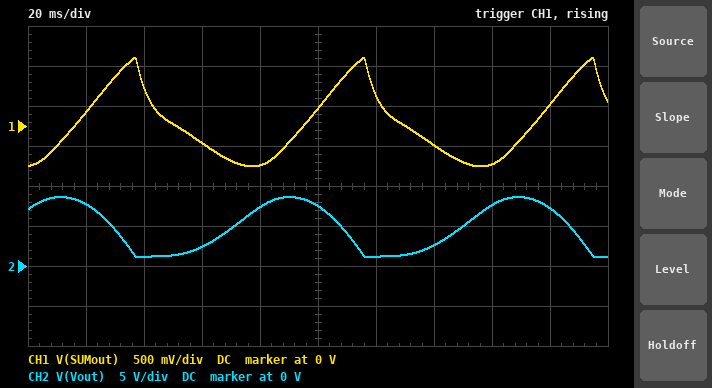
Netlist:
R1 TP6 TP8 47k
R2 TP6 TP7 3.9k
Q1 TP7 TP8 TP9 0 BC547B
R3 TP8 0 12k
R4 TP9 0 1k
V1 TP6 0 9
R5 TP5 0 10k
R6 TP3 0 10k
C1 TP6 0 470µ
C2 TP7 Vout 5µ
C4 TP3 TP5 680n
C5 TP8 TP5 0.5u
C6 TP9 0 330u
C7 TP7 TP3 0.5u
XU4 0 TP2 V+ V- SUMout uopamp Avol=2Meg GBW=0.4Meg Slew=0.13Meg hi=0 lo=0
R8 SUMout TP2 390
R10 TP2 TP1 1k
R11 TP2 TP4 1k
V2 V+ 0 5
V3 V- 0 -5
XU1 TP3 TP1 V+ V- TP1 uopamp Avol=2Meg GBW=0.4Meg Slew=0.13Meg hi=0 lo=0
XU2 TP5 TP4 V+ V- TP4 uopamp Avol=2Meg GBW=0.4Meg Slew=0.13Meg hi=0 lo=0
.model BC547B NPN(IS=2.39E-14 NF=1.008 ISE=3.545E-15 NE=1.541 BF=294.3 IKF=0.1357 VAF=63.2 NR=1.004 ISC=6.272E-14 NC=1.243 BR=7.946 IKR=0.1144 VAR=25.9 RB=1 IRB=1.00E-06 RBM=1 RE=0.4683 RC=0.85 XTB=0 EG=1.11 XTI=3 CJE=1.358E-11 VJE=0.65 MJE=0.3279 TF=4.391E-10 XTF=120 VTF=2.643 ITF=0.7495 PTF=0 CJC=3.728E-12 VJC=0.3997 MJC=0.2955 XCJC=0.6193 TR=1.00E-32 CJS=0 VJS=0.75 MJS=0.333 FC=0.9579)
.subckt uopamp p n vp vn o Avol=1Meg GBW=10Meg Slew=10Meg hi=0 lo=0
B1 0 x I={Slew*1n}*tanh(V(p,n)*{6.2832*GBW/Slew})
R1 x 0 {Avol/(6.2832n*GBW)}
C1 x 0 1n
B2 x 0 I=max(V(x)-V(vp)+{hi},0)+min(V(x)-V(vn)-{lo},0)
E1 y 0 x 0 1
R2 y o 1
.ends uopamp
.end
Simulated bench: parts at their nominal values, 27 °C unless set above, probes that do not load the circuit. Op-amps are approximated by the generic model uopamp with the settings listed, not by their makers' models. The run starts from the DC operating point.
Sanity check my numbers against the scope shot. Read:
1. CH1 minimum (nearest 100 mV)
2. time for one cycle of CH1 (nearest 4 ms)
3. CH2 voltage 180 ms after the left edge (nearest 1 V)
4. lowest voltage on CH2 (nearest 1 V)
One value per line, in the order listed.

-500 mV
80 ms
7 V
1 V
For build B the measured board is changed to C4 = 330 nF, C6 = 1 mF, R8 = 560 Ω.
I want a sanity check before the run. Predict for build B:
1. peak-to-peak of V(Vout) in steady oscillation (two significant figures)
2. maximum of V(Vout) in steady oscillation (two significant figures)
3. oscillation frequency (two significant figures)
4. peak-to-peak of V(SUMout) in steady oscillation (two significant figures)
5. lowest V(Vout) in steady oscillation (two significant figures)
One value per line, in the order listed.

7.1 V
8.3 V
14 Hz
2.0 V
1.2 V
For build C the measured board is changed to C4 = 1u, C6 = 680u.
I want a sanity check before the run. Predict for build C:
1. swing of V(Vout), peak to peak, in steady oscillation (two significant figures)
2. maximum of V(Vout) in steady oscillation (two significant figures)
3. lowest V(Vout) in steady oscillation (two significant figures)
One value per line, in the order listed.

7.1 V
8.3 V
1.2 V
